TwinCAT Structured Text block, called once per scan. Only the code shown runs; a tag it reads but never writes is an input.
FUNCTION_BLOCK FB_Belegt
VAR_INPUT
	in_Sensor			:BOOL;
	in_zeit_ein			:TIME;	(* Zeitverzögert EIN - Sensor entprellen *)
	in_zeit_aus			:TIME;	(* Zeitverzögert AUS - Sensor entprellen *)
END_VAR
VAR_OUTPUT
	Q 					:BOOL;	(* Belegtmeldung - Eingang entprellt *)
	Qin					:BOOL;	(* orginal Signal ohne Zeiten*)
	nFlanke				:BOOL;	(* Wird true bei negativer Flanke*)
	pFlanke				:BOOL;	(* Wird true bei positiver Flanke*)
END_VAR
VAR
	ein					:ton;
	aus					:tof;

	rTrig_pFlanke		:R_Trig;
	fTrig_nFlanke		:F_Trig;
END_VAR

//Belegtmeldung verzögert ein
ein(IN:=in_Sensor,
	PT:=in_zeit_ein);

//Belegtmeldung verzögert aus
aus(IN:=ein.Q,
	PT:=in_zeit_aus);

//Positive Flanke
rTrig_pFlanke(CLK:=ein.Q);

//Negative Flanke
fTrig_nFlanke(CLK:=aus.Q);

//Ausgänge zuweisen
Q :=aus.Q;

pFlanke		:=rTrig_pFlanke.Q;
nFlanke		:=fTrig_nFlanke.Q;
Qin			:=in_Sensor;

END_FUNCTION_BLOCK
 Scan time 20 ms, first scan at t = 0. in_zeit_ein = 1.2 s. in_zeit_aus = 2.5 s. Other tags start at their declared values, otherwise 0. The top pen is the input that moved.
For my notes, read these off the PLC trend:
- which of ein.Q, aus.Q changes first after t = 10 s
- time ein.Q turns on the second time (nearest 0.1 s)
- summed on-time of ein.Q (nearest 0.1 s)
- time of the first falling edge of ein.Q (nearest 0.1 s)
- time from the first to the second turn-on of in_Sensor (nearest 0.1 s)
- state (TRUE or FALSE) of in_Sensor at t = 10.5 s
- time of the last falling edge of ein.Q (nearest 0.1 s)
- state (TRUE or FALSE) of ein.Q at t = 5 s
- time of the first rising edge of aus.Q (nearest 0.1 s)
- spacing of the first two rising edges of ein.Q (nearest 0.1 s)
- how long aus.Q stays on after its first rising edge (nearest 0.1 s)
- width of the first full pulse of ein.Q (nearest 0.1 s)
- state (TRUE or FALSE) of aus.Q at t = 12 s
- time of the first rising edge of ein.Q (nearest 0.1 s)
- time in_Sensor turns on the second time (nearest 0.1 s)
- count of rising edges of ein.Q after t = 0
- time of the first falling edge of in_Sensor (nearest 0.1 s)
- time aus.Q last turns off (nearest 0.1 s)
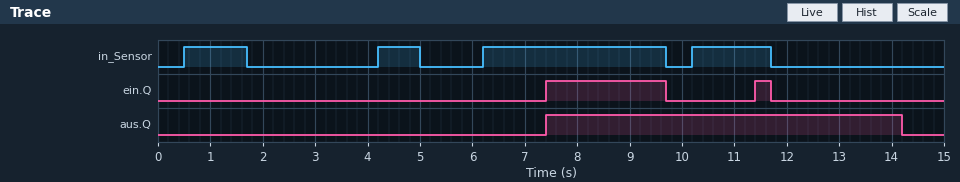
ein.Q
11.4 s
2.6 s
9.7 s
3.7 s
TRUE
11.7 s
FALSE
7.4 s
4.0 s
6.8 s
2.3 s
TRUE
7.4 s
4.2 s
2
1.7 s
14.2 s
